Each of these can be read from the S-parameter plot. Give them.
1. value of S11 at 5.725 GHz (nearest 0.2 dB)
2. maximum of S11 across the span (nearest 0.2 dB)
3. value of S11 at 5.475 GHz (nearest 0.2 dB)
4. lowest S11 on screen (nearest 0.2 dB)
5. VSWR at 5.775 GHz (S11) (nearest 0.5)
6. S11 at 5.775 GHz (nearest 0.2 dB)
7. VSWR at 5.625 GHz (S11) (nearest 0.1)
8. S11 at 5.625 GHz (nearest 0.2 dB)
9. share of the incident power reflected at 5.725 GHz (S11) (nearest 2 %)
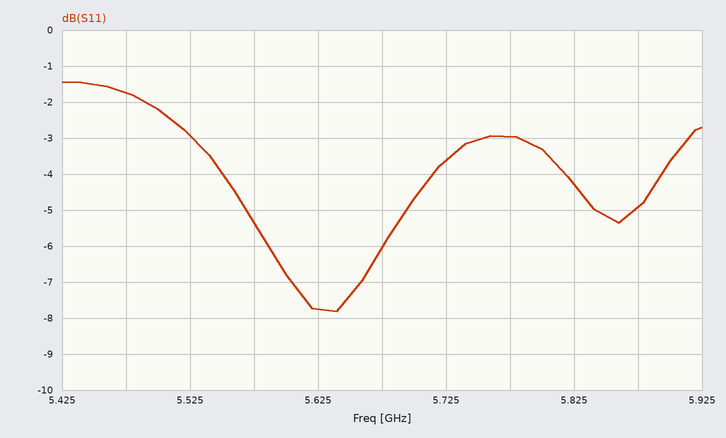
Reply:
-3.6 dB
-1.4 dB
-1.8 dB
-7.8 dB
6.0
-3.0 dB
2.4
-7.8 dB
44 %
